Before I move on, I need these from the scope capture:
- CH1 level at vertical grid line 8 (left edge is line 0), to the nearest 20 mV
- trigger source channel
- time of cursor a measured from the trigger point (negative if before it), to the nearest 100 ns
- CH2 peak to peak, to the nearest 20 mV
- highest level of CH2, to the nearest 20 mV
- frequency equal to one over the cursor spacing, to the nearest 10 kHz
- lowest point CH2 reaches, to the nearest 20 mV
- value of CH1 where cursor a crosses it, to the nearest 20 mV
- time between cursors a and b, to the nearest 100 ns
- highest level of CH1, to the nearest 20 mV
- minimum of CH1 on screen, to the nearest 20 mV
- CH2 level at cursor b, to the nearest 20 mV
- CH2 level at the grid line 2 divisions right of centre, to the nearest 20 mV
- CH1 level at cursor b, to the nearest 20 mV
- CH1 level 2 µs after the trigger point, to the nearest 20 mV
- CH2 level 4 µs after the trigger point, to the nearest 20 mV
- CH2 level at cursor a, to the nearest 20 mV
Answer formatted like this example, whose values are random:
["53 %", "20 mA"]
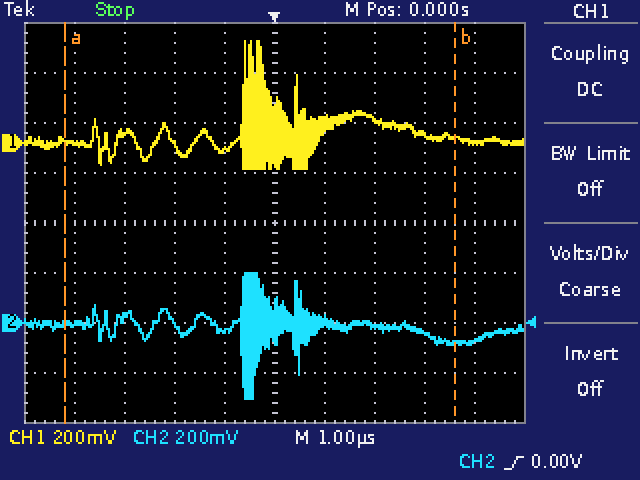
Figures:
["40 mV", "CH2", "-4.2 µs", "500 mV", "200 mV", "130 kHz", "-300 mV", "0 mV", "7.8 µs", "400 mV", "-100 mV", "-80 mV", "-20 mV", "20 mV", "100 mV", "-80 mV", "0 mV"]
